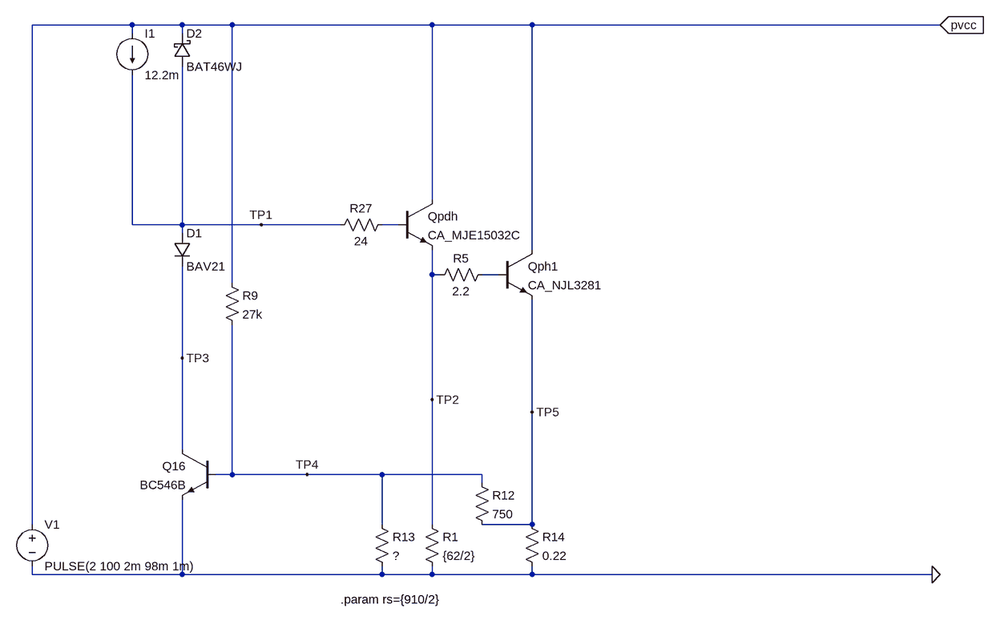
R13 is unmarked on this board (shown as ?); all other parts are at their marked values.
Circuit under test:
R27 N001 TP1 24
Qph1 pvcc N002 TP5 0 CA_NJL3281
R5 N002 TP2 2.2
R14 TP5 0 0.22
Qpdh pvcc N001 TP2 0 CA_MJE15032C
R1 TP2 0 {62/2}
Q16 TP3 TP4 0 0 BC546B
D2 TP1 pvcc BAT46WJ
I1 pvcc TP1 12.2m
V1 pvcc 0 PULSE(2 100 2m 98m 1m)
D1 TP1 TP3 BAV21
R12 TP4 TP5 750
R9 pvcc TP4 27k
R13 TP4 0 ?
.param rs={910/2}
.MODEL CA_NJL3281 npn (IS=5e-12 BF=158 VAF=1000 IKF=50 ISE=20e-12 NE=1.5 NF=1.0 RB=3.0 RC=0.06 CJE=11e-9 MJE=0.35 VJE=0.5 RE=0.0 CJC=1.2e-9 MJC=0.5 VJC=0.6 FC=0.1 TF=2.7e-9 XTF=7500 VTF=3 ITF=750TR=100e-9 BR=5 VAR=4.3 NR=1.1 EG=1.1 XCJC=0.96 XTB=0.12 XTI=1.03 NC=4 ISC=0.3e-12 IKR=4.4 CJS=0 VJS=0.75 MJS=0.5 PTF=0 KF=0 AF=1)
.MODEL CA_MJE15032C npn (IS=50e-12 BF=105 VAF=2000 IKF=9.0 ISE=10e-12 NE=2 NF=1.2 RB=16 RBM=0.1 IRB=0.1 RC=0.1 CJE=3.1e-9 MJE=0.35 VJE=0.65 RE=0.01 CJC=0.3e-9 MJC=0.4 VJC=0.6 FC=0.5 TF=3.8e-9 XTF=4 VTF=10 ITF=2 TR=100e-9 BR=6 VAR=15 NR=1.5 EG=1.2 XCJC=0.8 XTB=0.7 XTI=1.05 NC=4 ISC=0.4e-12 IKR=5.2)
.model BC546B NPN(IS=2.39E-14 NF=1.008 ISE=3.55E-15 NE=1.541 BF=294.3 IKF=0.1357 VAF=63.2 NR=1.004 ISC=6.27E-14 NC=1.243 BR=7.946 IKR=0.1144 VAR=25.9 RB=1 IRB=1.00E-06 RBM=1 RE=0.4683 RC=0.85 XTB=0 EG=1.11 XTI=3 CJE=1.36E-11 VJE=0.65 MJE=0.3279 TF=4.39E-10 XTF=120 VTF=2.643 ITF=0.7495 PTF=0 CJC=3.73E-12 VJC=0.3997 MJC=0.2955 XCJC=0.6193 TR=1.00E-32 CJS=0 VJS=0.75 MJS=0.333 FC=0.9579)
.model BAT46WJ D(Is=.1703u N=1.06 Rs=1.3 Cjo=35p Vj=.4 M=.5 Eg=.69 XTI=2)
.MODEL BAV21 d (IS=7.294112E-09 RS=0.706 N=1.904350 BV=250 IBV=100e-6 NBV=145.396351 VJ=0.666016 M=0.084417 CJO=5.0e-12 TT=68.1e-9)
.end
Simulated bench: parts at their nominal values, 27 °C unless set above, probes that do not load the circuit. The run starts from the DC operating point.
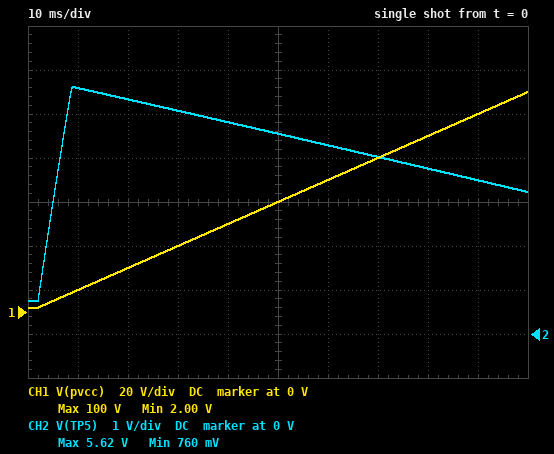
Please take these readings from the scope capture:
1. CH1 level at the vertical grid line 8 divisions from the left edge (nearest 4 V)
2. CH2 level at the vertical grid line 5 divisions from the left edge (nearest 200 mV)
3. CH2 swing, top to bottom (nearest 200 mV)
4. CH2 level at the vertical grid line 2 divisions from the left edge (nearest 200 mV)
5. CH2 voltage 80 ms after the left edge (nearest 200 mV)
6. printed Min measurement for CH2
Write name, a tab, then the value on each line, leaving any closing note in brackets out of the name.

CH1 level at the vertical grid line 8 divisions from the left edge	80 V
CH2 level at the vertical grid line 5 divisions from the left edge	4.6 V
CH2 swing, top to bottom	4.8 V
CH2 level at the vertical grid line 2 divisions from the left edge	5.4 V
CH2 voltage 80 ms after the left edge	3.8 V
printed Min measurement for CH2	760 mV
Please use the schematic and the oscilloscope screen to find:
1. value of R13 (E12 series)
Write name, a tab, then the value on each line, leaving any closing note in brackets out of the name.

value of R13	100 Ω
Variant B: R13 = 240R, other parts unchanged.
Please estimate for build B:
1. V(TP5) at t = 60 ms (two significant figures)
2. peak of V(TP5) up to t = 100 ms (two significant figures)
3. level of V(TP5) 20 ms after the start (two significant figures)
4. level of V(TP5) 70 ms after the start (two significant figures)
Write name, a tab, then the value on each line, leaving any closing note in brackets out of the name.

V(TP5) at t = 60 ms	1.3 V
peak of V(TP5) up to t = 100 ms	2.8 V
level of V(TP5) 20 ms after the start	2.4 V
level of V(TP5) 70 ms after the start	1.0 V
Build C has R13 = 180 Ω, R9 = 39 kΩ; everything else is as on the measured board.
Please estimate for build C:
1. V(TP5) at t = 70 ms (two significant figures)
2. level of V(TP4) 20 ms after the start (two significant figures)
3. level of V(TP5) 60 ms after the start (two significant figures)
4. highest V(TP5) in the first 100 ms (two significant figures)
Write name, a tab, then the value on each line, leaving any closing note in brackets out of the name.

V(TP5) at t = 70 ms	2.3 V
level of V(TP4) 20 ms after the start	700 mV
level of V(TP5) 60 ms after the start	2.5 V
highest V(TP5) in the first 100 ms	3.5 V
